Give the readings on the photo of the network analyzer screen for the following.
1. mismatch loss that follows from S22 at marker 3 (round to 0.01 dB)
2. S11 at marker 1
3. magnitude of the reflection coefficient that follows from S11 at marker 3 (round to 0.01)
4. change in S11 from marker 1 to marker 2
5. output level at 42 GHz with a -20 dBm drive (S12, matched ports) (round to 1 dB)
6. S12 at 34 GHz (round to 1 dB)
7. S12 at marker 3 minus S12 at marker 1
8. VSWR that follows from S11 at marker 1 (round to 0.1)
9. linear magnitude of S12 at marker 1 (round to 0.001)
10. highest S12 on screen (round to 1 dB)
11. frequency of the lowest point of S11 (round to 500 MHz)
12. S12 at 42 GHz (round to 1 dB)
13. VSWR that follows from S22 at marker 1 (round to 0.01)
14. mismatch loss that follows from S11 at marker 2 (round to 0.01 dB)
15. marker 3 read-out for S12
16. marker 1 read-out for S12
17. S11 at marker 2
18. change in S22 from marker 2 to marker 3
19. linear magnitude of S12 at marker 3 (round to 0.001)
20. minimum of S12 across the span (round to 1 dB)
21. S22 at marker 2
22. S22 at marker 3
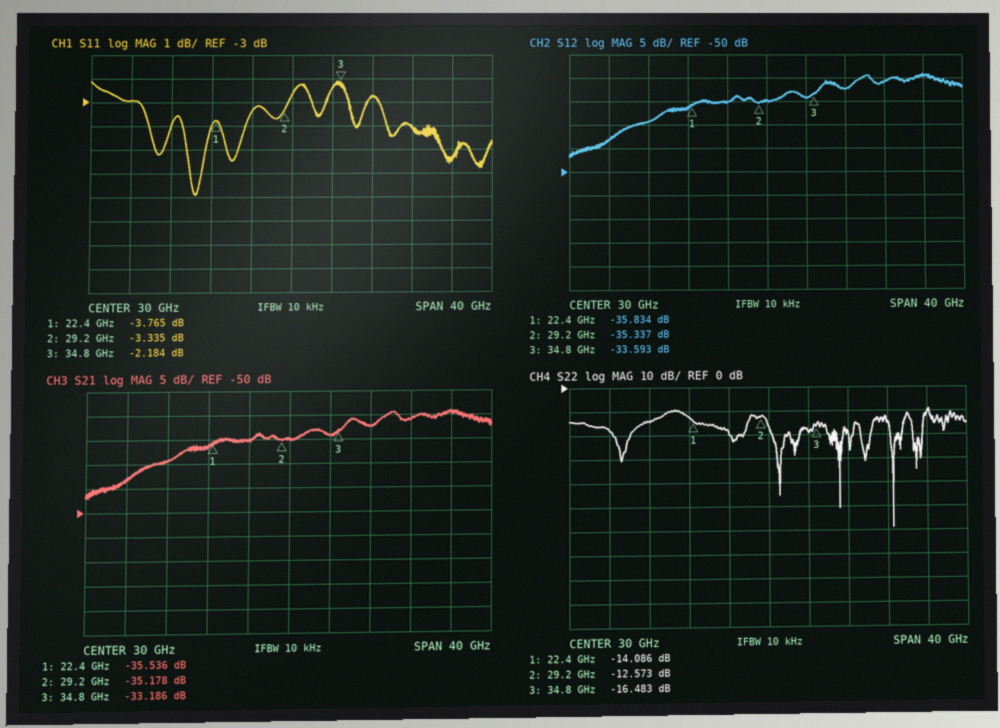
0.10 dB
-3.765 dB
0.78
0.430 dB
-51 dBm
-34 dB
2.241 dB
4.7
0.016
-29 dB
20.5 GHz
-31 dB
1.49
2.71 dB
-33.593 dB
-35.834 dB
-3.335 dB
-3.910 dB
0.021
-47 dB
-12.573 dB
-16.483 dB
